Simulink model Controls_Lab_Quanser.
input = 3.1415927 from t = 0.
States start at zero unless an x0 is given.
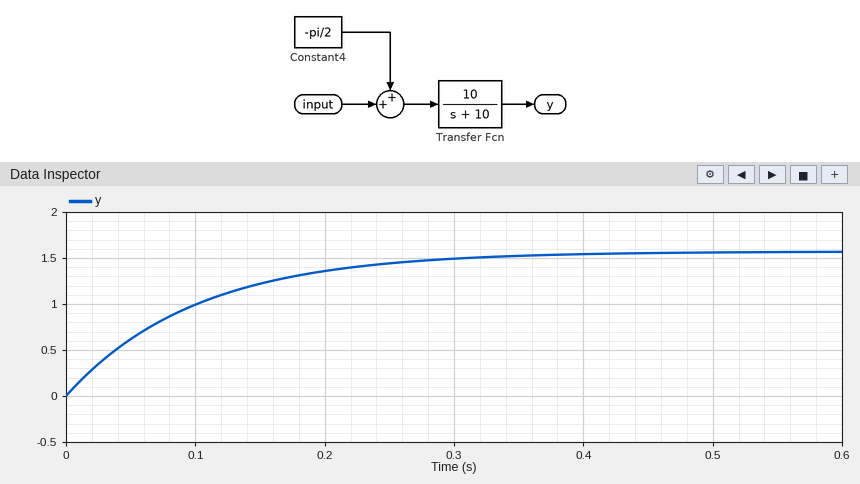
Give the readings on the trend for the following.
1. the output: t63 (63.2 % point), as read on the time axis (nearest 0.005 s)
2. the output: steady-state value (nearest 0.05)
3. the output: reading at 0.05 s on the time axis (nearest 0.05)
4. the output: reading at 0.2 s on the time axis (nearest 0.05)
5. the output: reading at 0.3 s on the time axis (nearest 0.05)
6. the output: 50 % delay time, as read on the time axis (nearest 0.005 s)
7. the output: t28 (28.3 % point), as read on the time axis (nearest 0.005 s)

0.100 s
1.55
0.60
1.35
1.50
0.070 s
0.035 s
